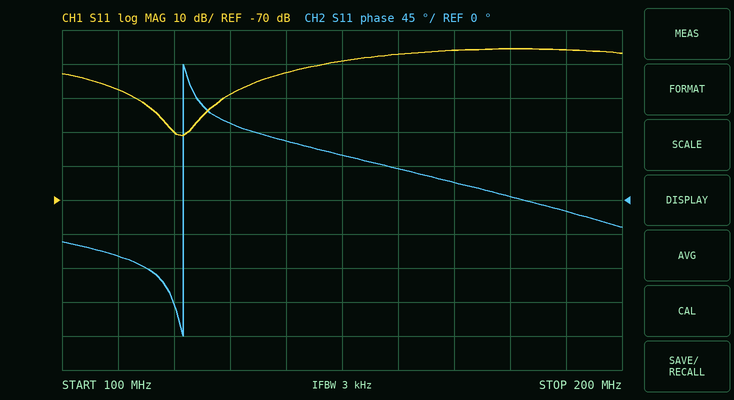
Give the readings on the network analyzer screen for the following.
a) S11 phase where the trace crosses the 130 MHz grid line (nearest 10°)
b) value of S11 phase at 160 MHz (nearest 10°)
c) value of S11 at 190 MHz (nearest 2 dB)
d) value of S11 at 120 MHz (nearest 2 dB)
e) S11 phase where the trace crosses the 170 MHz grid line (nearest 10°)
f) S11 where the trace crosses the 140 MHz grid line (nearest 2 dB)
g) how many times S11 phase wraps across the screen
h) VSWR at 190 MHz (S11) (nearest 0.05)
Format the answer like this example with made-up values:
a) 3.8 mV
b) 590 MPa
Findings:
a) 100°
b) 40°
c) -26 dB
d) -50 dB
e) 20°
f) -32 dB
g) 1
h) 1.10
